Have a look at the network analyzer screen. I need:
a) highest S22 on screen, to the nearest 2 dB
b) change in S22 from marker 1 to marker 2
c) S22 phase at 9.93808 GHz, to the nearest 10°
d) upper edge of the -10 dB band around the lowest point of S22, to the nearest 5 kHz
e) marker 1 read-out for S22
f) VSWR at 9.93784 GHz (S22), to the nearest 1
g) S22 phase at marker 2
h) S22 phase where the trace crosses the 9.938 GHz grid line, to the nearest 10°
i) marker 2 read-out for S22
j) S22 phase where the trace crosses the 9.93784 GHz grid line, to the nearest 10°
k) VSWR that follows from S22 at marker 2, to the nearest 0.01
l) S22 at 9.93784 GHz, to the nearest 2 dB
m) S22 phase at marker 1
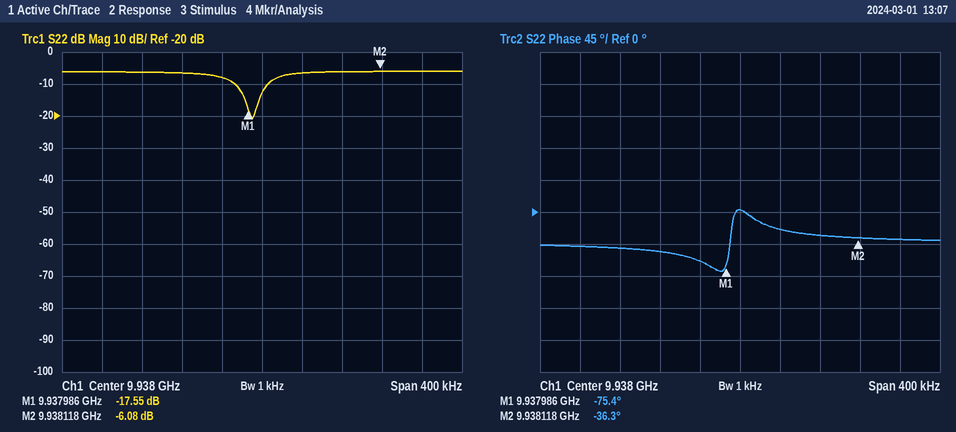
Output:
-6 dB
11.47 dB
-30°
9.938005 GHz
-17.55 dB
3
-36.3°
0°
-6.08 dB
-50°
2.97
-6 dB
-75.4°
